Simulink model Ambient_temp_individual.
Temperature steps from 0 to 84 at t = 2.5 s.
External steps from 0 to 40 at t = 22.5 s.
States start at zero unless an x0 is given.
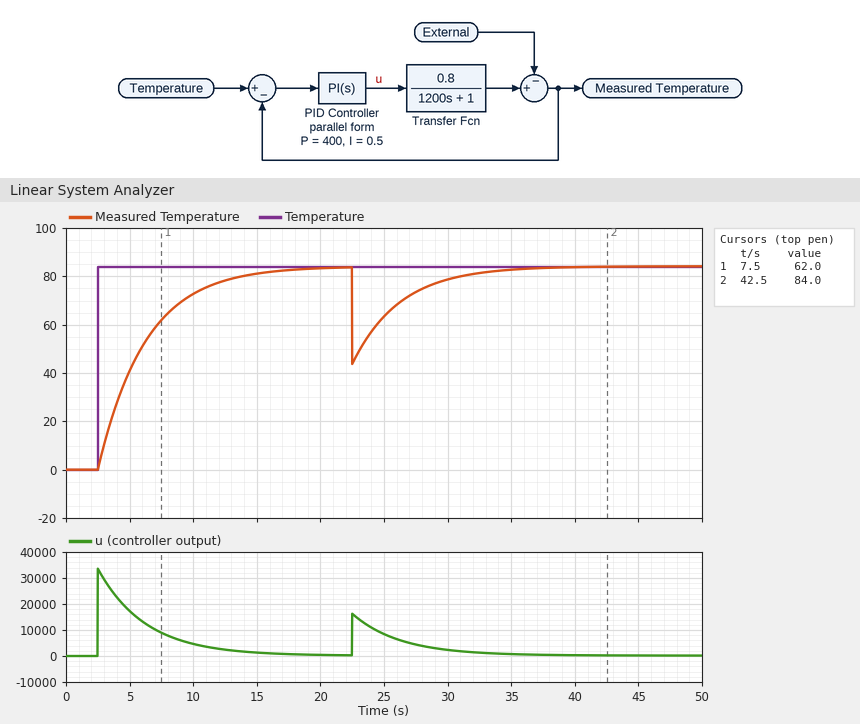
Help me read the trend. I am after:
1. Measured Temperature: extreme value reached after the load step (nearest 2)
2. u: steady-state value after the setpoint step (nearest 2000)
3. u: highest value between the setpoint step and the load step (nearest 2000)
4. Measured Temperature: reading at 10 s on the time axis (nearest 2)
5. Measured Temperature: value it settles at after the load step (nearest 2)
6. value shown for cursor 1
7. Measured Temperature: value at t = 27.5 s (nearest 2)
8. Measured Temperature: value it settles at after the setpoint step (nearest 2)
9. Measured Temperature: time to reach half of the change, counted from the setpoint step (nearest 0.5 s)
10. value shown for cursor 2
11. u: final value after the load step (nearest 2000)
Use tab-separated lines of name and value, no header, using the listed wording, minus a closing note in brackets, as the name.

Measured Temperature: extreme value reached after the load step	44
u: steady-state value after the setpoint step	0
u: highest value between the setpoint step and the load step	34000
Measured Temperature: reading at 10 s on the time axis	72
Measured Temperature: value it settles at after the load step	84
value shown for cursor 1	62.0
Measured Temperature: value at t = 27.5 s	74
Measured Temperature: value it settles at after the setpoint step	84
Measured Temperature: time to reach half of the change, counted from the setpoint step	2.5 s
value shown for cursor 2	84.0
u: final value after the load step	0
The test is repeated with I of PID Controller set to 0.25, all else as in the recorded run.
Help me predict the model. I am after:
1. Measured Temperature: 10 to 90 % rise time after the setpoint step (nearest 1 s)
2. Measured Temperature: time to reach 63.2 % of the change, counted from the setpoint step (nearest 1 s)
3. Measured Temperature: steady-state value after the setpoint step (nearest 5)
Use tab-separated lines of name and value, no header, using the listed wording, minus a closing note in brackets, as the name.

Measured Temperature: 10 to 90 % rise time after the setpoint step	8 s
Measured Temperature: time to reach 63.2 % of the change, counted from the setpoint step	4 s
Measured Temperature: steady-state value after the setpoint step	85
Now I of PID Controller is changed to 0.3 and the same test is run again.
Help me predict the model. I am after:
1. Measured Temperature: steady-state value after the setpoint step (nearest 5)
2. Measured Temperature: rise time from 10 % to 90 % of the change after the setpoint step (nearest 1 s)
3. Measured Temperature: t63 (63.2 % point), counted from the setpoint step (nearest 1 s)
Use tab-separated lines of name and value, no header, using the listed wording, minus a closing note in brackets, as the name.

Measured Temperature: steady-state value after the setpoint step	85
Measured Temperature: rise time from 10 % to 90 % of the change after the setpoint step	8 s
Measured Temperature: t63 (63.2 % point), counted from the setpoint step	4 s
